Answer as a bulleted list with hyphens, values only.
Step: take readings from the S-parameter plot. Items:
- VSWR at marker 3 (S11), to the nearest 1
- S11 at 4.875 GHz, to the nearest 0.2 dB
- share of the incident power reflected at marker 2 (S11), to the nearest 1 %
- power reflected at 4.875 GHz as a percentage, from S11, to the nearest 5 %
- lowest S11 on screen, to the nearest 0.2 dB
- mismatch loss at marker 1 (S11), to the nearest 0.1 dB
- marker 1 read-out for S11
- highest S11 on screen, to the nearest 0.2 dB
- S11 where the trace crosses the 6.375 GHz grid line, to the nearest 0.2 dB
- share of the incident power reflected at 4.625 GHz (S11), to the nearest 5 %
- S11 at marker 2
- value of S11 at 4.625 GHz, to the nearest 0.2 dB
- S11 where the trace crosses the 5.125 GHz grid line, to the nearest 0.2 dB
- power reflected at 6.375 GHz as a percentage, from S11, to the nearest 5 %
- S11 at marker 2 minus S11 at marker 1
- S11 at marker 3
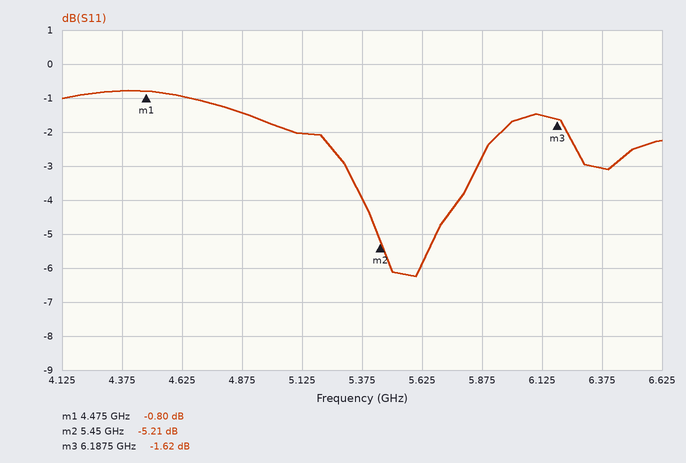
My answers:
- 11
- -1.4 dB
- 30 %
- 70 %
- -6.2 dB
- 7.7 dB
- -0.80 dB
- -0.8 dB
- -3.0 dB
- 80 %
- -5.21 dB
- -1.0 dB
- -2.0 dB
- 50 %
- -4.41 dB
- -1.62 dB
